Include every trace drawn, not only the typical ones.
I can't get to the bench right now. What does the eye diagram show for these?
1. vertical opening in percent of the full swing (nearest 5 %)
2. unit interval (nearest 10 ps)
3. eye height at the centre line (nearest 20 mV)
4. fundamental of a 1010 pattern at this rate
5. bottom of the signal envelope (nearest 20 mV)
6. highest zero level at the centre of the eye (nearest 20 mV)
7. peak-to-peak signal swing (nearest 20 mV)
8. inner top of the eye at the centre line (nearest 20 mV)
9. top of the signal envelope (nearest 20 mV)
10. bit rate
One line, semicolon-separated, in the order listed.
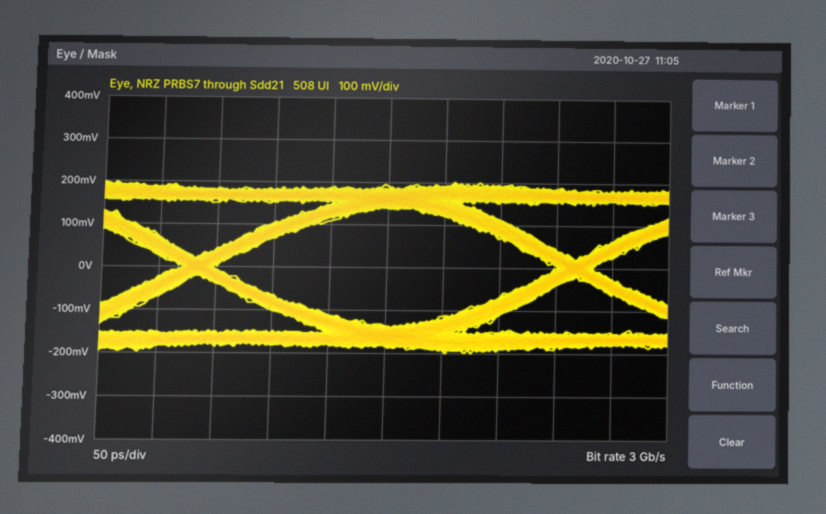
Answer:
70 %; 330 ps; 280 mV; 1.5 GHz; -200 mV; -140 mV; 400 mV; 140 mV; 200 mV; 3 Gb/s
